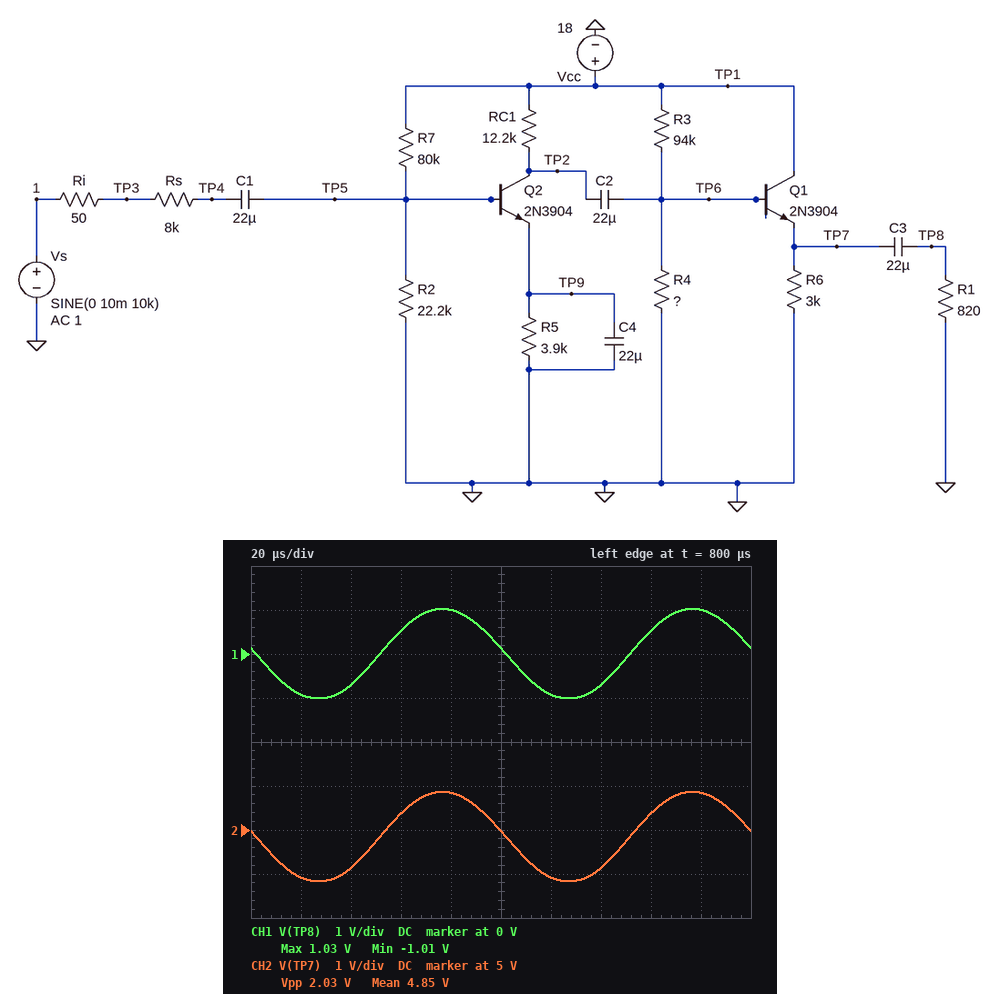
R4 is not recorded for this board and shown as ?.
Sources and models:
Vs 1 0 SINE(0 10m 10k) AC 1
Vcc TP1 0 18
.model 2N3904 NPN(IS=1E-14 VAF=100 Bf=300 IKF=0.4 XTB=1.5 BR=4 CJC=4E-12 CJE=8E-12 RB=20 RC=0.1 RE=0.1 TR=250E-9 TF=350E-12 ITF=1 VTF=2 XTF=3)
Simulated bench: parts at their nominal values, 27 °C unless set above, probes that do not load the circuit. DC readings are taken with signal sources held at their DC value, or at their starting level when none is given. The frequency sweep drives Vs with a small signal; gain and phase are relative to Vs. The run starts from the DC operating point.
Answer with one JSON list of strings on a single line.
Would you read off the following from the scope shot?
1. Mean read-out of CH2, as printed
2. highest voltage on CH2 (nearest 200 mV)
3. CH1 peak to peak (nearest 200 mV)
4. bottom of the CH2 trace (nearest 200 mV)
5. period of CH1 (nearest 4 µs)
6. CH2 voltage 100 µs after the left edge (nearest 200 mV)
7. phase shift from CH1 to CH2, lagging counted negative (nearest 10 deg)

["4.85 V", "5.8 V", "2.0 V", "3.8 V", "100 µs", "5.0 V", "0 deg"]
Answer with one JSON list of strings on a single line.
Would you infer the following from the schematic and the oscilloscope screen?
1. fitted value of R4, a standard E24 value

["43 kΩ"]
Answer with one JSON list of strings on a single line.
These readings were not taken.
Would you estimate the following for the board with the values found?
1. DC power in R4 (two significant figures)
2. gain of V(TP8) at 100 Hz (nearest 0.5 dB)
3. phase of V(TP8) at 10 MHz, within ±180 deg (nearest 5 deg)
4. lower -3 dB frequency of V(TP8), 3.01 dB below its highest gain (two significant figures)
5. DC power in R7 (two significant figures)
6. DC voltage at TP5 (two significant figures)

["710 µW", "35.5 dB", "85 deg", "140 Hz", "2.5 mW", "3.9 V"]
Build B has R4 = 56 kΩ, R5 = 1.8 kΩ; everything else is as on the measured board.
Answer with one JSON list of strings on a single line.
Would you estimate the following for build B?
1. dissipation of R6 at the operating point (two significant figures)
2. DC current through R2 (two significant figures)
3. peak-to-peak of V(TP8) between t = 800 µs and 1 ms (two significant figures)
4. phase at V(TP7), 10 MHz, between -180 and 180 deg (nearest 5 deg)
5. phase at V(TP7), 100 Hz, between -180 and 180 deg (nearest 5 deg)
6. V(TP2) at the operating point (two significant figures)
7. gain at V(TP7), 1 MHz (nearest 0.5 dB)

["11 mW", "140 µA", "1.2 mV", "25 deg", "-170 deg", "2.4 V", "-40.5 dB"]
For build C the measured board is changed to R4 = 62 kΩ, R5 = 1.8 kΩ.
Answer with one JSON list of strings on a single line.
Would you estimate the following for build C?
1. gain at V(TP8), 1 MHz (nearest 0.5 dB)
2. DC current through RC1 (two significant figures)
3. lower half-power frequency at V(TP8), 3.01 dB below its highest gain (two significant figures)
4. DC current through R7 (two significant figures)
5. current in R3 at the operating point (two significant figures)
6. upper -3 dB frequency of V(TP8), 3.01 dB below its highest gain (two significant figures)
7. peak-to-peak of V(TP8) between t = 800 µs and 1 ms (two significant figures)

["-40.5 dB", "1.3 mA", "4.8 Hz", "190 µA", "120 µA", "160 kHz", "1.2 mV"]
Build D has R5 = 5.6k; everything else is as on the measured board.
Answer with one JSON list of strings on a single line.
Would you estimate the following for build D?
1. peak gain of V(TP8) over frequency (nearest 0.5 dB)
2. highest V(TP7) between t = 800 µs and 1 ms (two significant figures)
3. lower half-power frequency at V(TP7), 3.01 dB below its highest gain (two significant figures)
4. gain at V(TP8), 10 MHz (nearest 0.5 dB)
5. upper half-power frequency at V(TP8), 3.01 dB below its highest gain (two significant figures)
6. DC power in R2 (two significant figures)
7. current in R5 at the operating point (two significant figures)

["38.5 dB", "5.7 V", "110 Hz", "-0.5 dB", "110 kHz", "680 µW", "580 µA"]
